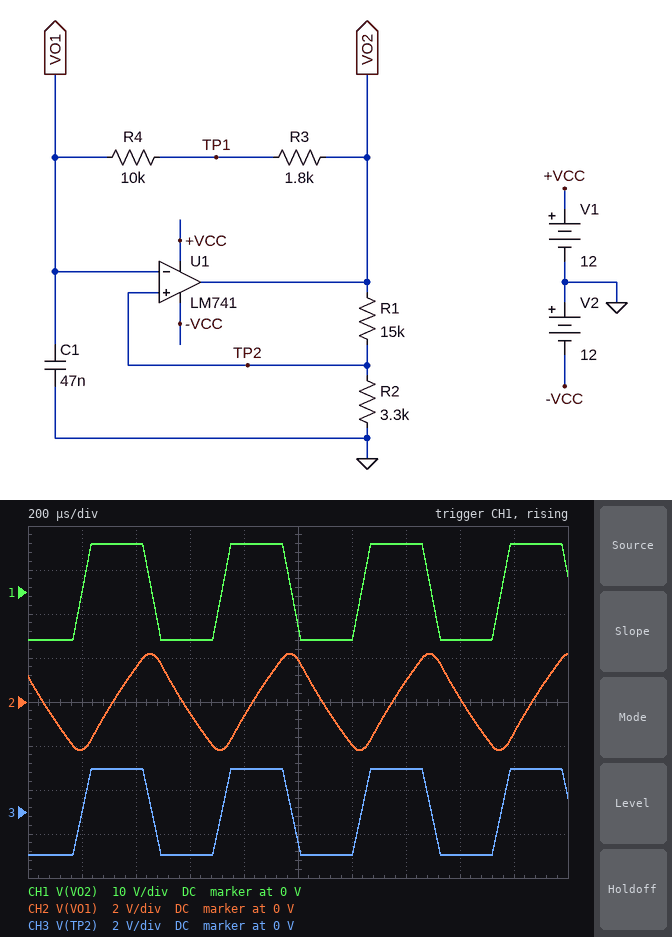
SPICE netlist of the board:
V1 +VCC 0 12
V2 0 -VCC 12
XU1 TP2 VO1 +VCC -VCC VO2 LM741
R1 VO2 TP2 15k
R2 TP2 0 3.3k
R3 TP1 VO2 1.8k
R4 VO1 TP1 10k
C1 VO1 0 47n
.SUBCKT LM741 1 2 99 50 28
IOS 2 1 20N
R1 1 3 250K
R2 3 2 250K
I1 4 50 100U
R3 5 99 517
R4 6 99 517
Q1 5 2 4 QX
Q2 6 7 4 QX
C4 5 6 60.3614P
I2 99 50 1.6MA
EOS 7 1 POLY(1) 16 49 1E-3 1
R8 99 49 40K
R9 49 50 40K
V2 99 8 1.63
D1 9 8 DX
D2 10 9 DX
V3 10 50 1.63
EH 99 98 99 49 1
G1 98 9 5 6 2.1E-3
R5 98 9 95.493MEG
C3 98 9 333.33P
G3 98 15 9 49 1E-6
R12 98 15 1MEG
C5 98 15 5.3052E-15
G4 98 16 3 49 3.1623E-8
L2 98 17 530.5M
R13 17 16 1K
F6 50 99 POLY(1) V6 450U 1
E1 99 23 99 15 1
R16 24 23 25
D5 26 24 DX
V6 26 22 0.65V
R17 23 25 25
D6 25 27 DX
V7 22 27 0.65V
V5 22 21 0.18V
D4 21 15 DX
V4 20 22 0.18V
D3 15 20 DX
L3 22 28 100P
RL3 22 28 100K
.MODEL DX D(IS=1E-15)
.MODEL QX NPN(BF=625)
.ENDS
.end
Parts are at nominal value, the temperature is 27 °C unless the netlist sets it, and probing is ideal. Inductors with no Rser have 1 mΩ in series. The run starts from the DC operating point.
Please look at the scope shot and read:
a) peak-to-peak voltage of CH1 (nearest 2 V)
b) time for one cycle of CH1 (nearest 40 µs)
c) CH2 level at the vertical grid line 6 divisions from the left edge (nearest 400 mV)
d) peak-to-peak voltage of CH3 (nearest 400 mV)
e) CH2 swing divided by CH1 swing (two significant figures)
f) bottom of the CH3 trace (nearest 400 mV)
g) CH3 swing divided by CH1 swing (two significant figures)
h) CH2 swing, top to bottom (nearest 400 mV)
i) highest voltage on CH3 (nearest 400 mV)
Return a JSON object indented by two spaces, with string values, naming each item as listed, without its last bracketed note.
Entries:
{
  "peak-to-peak voltage of CH1": "22 V",
  "time for one cycle of CH1": "520 µs",
  "CH2 level at the vertical grid line 6 divisions from the left edge": "-2.0 V",
  "peak-to-peak voltage of CH3": "4.0 V",
  "CH2 swing divided by CH1 swing": "0.20",
  "bottom of the CH3 trace": "-2.0 V",
  "CH3 swing divided by CH1 swing": "0.18",
  "CH2 swing, top to bottom": "4.4 V",
  "highest voltage on CH3": "2.0 V"
}
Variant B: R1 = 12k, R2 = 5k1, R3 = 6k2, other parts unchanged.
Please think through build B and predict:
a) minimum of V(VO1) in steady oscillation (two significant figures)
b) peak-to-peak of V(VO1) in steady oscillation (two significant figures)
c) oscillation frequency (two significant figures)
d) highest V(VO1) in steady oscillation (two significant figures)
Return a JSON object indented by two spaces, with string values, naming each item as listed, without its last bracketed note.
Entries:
{
  "minimum of V(VO1) in steady oscillation": "-3.4 V",
  "peak-to-peak of V(VO1) in steady oscillation": "6.7 V",
  "oscillation frequency": "970 Hz",
  "highest V(VO1) in steady oscillation": "3.4 V"
}
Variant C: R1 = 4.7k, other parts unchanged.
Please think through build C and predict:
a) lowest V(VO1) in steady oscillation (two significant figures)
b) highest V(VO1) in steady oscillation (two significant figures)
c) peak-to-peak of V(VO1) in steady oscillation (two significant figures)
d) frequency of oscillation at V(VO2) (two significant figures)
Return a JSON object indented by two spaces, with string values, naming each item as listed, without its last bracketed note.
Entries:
{
  "lowest V(VO1) in steady oscillation": "-4.6 V",
  "highest V(VO1) in steady oscillation": "4.6 V",
  "peak-to-peak of V(VO1) in steady oscillation": "9.2 V",
  "frequency of oscillation at V(VO2)": "940 Hz"
}
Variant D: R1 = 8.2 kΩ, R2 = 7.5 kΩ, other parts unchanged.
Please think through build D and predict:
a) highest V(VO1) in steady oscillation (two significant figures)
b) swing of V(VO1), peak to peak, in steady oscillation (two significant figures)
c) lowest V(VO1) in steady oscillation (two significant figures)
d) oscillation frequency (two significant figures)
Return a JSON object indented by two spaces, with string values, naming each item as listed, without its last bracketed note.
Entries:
{
  "highest V(VO1) in steady oscillation": "5.3 V",
  "swing of V(VO1), peak to peak, in steady oscillation": "11 V",
  "lowest V(VO1) in steady oscillation": "-5.3 V",
  "oscillation frequency": "810 Hz"
}
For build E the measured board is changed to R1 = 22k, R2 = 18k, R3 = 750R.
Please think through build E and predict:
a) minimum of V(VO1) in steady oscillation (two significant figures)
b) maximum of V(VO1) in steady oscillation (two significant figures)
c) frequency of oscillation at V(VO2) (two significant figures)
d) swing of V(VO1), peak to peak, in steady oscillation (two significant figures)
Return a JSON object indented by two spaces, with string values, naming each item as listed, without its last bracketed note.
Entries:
{
  "minimum of V(VO1) in steady oscillation": "-5.0 V",
  "maximum of V(VO1) in steady oscillation": "5.0 V",
  "frequency of oscillation at V(VO2)": "940 Hz",
  "swing of V(VO1), peak to peak, in steady oscillation": "10 V"
}
